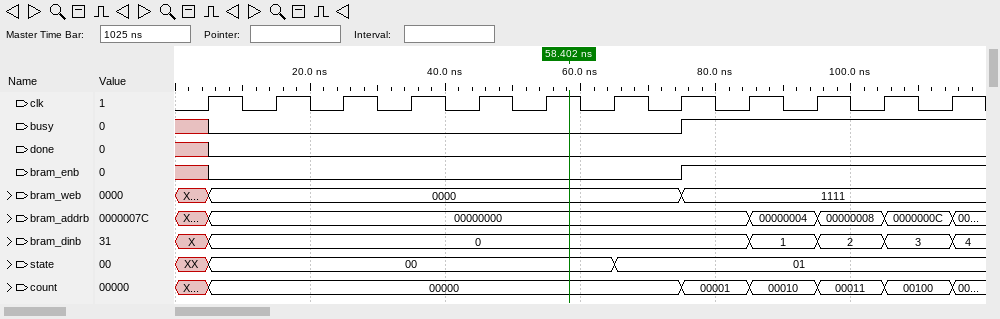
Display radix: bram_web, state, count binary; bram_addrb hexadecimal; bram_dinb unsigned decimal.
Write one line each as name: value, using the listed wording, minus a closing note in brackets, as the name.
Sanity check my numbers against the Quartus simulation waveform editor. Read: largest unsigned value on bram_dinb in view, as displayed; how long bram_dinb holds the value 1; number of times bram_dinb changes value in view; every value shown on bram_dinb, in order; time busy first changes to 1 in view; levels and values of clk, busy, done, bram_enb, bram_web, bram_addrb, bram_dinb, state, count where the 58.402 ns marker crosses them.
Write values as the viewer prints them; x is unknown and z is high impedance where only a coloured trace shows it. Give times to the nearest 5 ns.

largest unsigned value on bram_dinb in view, as displayed: 4
how long bram_dinb holds the value 1: 10 ns
number of times bram_dinb changes value in view: 5
every value shown on bram_dinb, in order: X, 0, 1, 2, 3, 4
time busy first changes to 1 in view: 75 ns
levels and values of clk, busy, done, bram_enb, bram_web, bram_addrb, bram_dinb, state, count where the 58.402 ns marker crosses them: clk=1, busy=0, done=0, bram_enb=0, bram_web=0000, bram_addrb=00000000, bram_dinb=0, state=00, count=00000
